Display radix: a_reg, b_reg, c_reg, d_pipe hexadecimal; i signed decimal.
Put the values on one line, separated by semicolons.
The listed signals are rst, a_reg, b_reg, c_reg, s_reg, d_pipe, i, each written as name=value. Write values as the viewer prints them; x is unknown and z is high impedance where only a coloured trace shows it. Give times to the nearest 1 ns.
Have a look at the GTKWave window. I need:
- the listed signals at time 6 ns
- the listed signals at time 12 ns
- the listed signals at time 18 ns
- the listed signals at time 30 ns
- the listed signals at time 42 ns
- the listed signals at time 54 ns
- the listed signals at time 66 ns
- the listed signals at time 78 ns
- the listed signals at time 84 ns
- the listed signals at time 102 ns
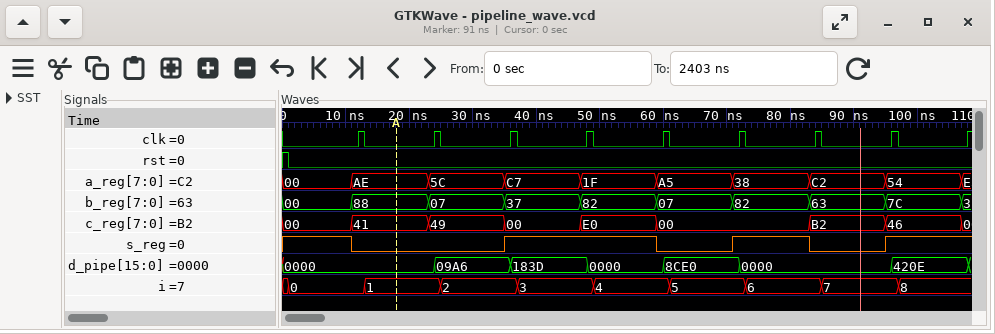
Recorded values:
rst=0, a_reg=00, b_reg=00, c_reg=00, s_reg=1, d_pipe=0000, i=0; rst=0, a_reg=AE, b_reg=88, c_reg=41, s_reg=0, d_pipe=0000, i=0; rst=0, a_reg=AE, b_reg=88, c_reg=41, s_reg=0, d_pipe=0000, i=1; rst=0, a_reg=5C, b_reg=07, c_reg=49, s_reg=0, d_pipe=09A6, i=2; rst=0, a_reg=C7, b_reg=37, c_reg=00, s_reg=1, d_pipe=183D, i=3; rst=0, a_reg=1F, b_reg=82, c_reg=E0, s_reg=1, d_pipe=0000, i=4; rst=0, a_reg=A5, b_reg=07, c_reg=00, s_reg=0, d_pipe=8CE0, i=5; rst=0, a_reg=38, b_reg=82, c_reg=00, s_reg=1, d_pipe=0000, i=6; rst=0, a_reg=C2, b_reg=63, c_reg=B2, s_reg=0, d_pipe=0000, i=6; rst=0, a_reg=54, b_reg=7C, c_reg=46, s_reg=1, d_pipe=420E, i=8
